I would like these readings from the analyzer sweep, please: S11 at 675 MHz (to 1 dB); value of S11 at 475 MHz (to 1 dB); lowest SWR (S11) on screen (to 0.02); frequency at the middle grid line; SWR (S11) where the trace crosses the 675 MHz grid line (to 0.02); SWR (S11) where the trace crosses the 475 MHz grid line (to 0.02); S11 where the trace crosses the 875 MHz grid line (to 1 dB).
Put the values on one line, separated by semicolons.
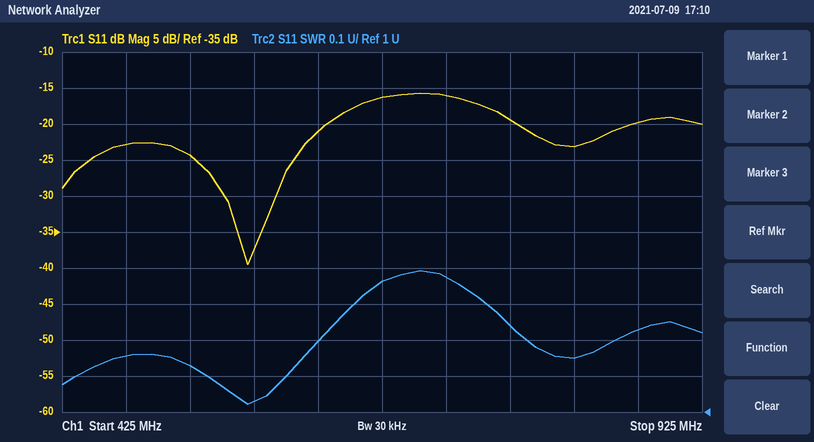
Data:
-16 dB; -23 dB; 1.02; 675 MHz; 1.36; 1.16; -20 dB
